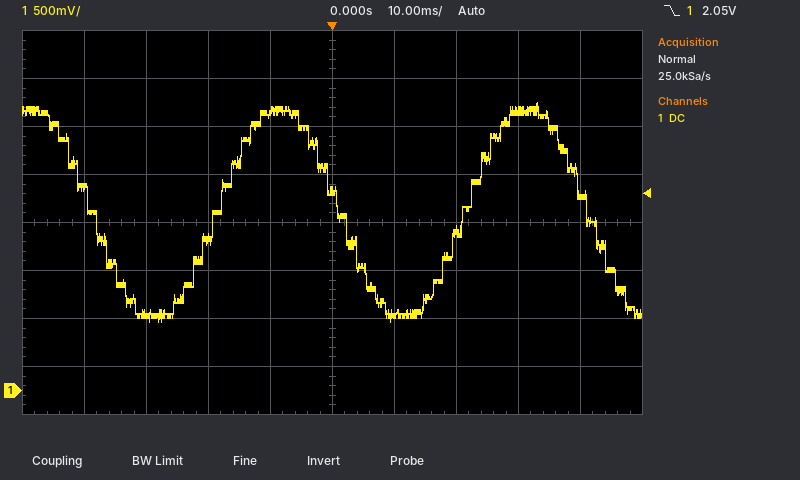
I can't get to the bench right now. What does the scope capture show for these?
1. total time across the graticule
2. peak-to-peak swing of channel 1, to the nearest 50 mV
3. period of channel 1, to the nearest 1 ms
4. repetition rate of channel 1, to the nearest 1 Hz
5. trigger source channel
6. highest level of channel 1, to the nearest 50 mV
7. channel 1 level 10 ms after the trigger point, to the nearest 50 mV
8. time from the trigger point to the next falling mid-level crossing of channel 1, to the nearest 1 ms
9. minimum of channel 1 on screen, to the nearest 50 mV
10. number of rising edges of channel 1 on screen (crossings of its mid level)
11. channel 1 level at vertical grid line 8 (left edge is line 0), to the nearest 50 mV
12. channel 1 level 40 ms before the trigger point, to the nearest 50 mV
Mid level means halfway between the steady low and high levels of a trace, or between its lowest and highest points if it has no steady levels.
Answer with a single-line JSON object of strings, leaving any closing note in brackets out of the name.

{"total time across the graticule": "100 ms", "peak-to-peak swing of channel 1, to the nearest 50 mV": "2.30 V", "period of channel 1, to the nearest 1 ms": "40 ms", "repetition rate of channel 1, to the nearest 1 Hz": "25 Hz", "trigger source channel": "channel 1", "highest level of channel 1, to the nearest 50 mV": "3.00 V", "channel 1 level 10 ms after the trigger point, to the nearest 50 mV": "800 mV", "time from the trigger point to the next falling mid-level crossing of channel 1, to the nearest 1 ms": "1 ms", "minimum of channel 1 on screen, to the nearest 50 mV": "700 mV", "number of rising edges of channel 1 on screen": "2", "channel 1 level at vertical grid line 8 (left edge is line 0), to the nearest 50 mV": "2.90 V", "channel 1 level 40 ms before the trigger point, to the nearest 50 mV": "2.10 V"}
